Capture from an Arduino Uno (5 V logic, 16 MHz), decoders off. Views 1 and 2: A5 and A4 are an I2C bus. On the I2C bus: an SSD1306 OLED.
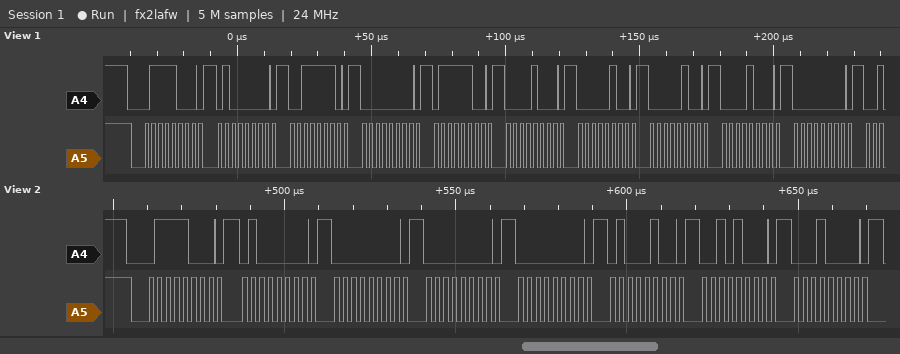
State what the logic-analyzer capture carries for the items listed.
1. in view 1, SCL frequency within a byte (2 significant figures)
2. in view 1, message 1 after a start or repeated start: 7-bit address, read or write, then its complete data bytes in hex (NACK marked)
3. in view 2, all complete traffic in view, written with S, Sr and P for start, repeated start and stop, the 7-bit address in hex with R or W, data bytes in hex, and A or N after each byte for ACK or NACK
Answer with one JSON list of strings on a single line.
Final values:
["400 kHz", "0x3C write: 40 3E 00 7C 08 04 04 08 00", "S 3CW A 40 A 00 A 00 A 00 A 44 A 28 A 10 A"]
